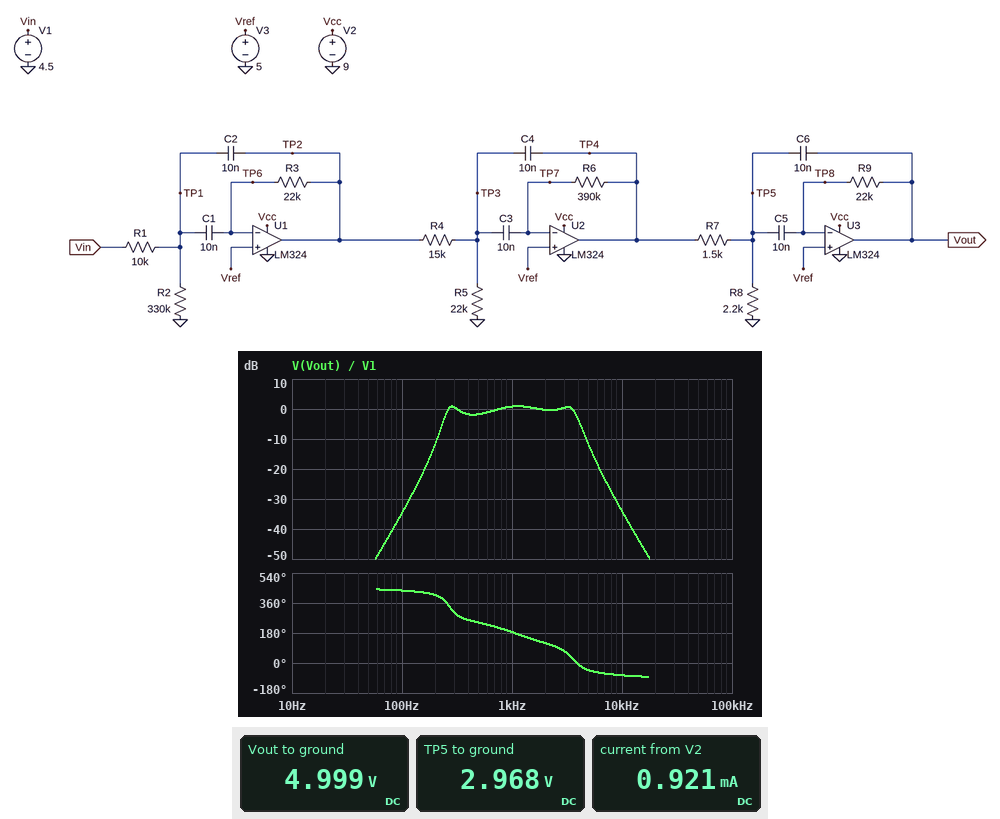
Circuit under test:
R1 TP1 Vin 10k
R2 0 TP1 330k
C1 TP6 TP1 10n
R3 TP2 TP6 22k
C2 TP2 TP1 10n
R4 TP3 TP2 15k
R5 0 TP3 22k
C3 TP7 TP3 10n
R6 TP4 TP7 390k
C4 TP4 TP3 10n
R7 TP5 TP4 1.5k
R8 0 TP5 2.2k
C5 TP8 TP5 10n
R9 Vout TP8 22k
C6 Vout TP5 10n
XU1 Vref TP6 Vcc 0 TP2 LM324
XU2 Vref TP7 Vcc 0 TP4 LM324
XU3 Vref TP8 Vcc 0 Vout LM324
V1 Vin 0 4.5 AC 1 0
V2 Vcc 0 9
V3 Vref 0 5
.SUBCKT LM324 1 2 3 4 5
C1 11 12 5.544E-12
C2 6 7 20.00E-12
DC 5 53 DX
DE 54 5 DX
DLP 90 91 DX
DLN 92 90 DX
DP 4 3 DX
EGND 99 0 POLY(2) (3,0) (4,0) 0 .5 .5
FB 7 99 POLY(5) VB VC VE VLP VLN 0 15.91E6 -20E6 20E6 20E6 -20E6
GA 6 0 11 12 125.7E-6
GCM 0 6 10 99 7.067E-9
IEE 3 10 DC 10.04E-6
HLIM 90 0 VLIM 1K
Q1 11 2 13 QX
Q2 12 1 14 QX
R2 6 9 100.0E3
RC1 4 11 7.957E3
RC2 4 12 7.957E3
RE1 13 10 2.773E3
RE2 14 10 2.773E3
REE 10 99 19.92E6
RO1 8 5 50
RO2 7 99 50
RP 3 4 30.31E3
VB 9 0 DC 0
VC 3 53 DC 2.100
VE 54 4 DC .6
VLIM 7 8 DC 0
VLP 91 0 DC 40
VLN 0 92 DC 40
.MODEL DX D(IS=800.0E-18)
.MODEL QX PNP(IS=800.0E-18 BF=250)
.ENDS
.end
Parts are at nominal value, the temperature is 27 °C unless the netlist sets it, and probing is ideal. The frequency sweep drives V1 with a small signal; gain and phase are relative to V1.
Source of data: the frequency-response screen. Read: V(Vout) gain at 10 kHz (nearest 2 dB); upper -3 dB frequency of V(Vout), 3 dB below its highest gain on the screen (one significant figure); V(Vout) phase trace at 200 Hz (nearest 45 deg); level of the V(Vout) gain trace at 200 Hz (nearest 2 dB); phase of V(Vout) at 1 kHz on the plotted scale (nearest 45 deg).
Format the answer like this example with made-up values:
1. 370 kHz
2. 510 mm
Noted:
1. -34 dB
2. 4 kHz
3. 405 deg
4. -12 dB
5. 180 deg
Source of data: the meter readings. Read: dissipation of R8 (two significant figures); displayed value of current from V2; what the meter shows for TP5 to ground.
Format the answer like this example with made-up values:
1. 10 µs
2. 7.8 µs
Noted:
1. 4.0 mW
2. 0.921 mA
3. 2.968 V
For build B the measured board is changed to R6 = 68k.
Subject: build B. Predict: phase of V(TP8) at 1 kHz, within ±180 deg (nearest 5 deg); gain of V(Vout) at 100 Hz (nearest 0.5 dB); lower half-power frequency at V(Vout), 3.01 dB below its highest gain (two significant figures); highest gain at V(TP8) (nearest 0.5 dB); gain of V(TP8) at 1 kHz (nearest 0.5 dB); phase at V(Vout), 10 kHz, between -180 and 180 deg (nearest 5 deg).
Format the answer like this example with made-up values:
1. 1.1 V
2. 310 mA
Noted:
1. 130 deg
2. -51.0 dB
3. 620 Hz
4. -48.5 dB
5. -57.0 dB
6. -70 deg
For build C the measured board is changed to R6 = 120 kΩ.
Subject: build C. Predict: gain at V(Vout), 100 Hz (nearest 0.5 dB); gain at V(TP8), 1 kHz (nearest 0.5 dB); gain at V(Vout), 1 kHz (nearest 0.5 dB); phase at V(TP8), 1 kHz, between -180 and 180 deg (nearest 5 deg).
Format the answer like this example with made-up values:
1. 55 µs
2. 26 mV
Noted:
1. -46.0 dB
2. -58.0 dB
3. 2.0 dB
4. 110 deg
